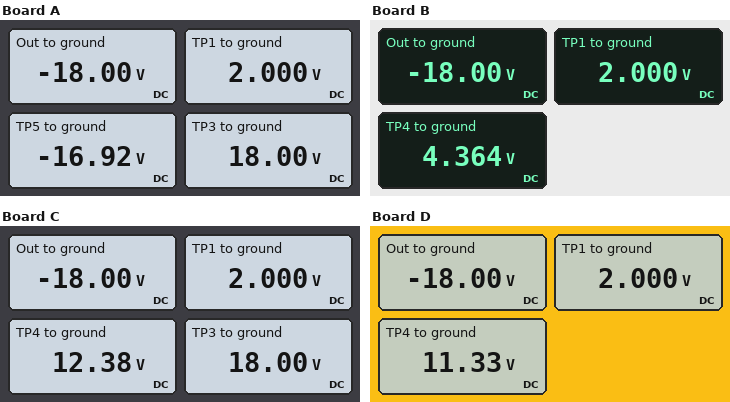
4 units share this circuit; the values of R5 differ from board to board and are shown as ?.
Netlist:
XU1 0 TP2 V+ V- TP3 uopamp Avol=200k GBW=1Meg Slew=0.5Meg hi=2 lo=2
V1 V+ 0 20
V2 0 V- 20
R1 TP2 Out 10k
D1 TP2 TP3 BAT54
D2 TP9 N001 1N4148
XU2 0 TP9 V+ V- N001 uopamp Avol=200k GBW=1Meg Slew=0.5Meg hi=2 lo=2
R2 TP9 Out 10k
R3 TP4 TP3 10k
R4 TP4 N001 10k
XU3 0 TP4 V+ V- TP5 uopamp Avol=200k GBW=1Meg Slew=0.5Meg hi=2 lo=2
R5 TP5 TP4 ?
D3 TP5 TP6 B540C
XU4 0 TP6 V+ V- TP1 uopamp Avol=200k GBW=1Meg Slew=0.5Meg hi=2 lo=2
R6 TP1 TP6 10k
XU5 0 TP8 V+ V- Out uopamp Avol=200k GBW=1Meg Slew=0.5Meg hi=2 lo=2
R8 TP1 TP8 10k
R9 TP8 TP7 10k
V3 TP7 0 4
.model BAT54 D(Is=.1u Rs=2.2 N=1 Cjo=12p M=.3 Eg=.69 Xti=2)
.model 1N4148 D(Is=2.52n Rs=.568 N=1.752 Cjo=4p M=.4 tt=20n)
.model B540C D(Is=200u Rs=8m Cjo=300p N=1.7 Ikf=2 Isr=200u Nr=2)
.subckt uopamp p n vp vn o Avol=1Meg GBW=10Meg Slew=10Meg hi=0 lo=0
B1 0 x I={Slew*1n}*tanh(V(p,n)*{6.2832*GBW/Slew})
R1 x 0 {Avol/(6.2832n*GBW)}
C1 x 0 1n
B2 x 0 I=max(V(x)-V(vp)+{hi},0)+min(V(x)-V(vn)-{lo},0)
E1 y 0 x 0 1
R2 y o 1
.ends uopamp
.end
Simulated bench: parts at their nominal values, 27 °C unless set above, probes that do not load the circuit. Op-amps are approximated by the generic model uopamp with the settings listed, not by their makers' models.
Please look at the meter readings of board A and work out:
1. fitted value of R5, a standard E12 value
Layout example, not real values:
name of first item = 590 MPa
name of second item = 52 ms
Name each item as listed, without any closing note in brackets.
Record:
fitted value of R5, a standard E12 value = 4.7 kΩ
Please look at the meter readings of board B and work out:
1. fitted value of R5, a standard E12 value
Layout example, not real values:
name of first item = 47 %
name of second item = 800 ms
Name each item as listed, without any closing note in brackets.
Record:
fitted value of R5, a standard E12 value = 8.2 kΩ
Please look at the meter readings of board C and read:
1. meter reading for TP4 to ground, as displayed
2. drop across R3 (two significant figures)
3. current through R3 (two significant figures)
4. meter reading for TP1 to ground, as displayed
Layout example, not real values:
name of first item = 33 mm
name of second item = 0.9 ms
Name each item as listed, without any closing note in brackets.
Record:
meter reading for TP4 to ground, as displayed = 12.38 V
drop across R3 = 5.6 V
current through R3 = 560 µA
meter reading for TP1 to ground, as displayed = 2.000 V
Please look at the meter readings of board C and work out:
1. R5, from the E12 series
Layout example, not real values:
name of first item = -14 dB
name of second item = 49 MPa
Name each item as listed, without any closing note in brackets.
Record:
R5, from the E12 series = 27 kΩ
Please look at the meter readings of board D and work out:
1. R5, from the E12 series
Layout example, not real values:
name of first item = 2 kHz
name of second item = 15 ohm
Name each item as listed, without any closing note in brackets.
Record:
R5, from the E12 series = 22 kΩ
